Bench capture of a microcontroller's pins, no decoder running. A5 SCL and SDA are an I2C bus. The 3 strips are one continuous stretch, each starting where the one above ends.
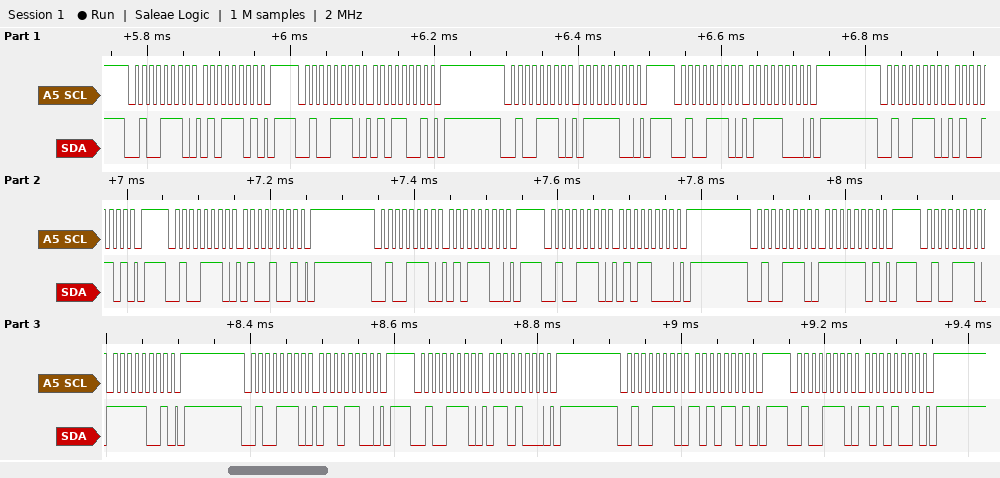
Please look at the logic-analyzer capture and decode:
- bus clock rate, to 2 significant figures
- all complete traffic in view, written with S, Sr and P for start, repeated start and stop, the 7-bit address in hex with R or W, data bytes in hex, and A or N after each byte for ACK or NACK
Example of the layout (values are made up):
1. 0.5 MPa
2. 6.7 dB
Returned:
1. 100 kHz
2. S 27W A 5D A P S 27W A 59 A P S 27W A 7C A P S 27W A 78 A P S 27W A 4D A P S 27W A 49 A P S 27W A 5C A P S 27W A 58 A P S 27W A FD A P S 27W A F9 A P S 27W A 6C A P S 27W A 68 A P S 27W A AD A P S 27W A A9 A P
